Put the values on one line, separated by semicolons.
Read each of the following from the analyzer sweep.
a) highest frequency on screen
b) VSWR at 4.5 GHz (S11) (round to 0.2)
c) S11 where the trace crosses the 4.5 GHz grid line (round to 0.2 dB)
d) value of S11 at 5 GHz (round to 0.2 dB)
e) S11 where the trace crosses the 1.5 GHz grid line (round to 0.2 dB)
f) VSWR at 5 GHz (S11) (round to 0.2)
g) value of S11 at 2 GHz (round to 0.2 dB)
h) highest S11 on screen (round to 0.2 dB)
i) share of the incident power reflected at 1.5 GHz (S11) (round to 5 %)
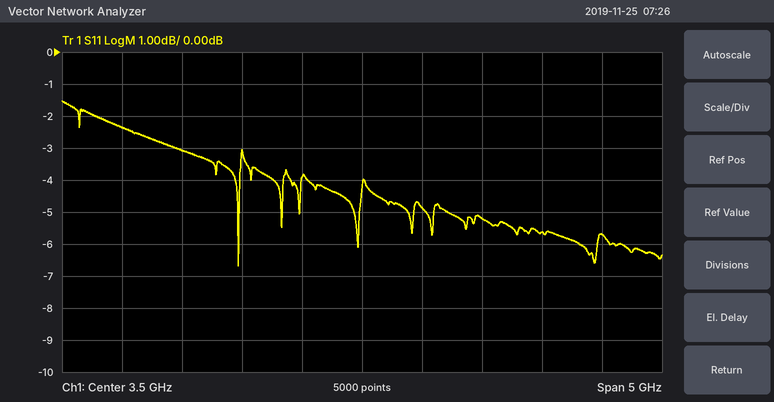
6 GHz; 3.4; -5.2 dB; -5.6 dB; -2.4 dB; 3.2; -3.0 dB; -1.6 dB; 60 %
